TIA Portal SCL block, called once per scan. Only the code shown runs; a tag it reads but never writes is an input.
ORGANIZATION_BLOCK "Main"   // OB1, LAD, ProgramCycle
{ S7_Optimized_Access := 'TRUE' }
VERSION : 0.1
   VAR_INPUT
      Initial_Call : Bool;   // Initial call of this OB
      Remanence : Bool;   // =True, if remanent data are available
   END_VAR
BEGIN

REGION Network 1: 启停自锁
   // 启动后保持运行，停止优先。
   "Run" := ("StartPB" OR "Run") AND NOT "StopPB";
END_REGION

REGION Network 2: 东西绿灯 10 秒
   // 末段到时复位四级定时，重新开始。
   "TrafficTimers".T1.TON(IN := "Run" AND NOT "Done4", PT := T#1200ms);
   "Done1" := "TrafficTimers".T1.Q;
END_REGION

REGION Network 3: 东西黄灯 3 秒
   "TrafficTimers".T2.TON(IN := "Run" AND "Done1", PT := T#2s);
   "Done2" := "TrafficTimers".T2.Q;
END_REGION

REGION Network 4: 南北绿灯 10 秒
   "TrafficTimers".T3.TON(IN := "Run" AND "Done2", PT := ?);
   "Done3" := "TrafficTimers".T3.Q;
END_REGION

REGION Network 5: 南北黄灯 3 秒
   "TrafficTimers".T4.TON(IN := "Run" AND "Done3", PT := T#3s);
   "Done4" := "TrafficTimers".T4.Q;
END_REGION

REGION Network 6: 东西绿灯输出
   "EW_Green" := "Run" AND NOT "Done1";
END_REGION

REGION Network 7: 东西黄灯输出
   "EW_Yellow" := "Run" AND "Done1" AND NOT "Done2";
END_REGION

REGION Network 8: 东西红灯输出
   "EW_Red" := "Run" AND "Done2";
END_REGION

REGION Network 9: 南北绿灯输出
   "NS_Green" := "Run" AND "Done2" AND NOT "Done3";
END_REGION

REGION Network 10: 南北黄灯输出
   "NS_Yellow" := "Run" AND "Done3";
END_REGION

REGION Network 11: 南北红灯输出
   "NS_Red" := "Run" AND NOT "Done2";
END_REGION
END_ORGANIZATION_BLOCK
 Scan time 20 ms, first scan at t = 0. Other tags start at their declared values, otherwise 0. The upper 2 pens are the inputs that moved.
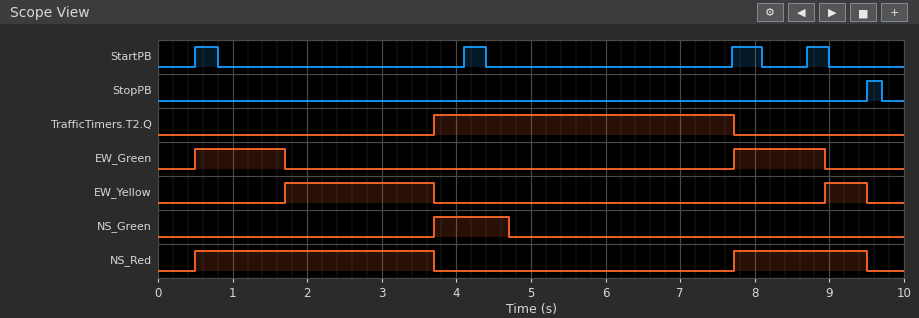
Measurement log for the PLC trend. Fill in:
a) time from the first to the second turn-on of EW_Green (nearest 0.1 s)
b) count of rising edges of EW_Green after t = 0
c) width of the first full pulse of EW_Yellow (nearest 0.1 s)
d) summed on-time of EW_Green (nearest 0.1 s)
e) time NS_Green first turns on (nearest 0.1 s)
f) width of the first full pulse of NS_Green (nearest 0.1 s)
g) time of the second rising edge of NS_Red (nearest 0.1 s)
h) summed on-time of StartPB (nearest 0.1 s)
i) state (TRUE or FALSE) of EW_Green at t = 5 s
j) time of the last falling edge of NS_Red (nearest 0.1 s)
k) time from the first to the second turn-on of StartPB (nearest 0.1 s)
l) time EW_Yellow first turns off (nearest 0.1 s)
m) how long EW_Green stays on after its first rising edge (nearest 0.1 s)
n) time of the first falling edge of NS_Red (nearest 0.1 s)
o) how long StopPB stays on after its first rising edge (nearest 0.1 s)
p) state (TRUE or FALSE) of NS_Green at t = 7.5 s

7.2 s
2
2.0 s
2.4 s
3.7 s
1.0 s
7.7 s
1.3 s
FALSE
9.5 s
3.6 s
3.7 s
1.2 s
3.7 s
0.2 s
FALSE
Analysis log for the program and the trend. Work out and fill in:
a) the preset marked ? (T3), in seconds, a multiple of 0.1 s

1.0 s
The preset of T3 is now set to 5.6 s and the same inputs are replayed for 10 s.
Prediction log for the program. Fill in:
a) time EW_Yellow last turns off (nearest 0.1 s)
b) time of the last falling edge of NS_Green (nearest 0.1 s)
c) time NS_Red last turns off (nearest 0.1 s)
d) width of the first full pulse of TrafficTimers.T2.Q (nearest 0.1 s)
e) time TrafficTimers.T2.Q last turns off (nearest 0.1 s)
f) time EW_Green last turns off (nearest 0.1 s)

3.7 s
9.3 s
3.7 s
5.8 s
9.5 s
1.7 s
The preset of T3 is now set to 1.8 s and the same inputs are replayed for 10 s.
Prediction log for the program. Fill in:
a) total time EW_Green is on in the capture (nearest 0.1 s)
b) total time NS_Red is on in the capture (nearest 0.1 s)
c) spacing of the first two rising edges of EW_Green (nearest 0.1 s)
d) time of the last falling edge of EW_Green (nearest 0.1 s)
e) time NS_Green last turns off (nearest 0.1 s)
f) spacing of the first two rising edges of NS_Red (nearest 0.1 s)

2.2 s
4.2 s
8.0 s
9.5 s
5.5 s
8.0 s
